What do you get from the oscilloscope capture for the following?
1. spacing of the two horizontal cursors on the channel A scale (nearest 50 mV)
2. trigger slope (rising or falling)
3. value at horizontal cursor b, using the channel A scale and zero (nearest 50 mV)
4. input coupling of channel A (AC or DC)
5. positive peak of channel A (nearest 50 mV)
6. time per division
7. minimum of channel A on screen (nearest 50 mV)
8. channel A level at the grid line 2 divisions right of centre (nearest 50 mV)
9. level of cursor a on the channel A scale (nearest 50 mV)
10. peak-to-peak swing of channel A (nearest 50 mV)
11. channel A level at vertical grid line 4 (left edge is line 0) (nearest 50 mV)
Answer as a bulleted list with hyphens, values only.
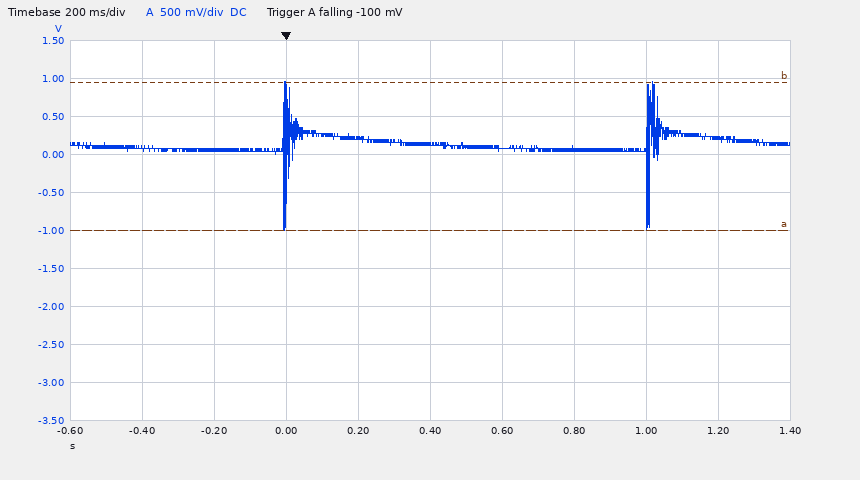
- 1.95 V
- falling
- 950 mV
- DC
- 950 mV
- 200 ms
- -1.00 V
- 100 mV
- -1.00 V
- 1.95 V
- 200 mV
